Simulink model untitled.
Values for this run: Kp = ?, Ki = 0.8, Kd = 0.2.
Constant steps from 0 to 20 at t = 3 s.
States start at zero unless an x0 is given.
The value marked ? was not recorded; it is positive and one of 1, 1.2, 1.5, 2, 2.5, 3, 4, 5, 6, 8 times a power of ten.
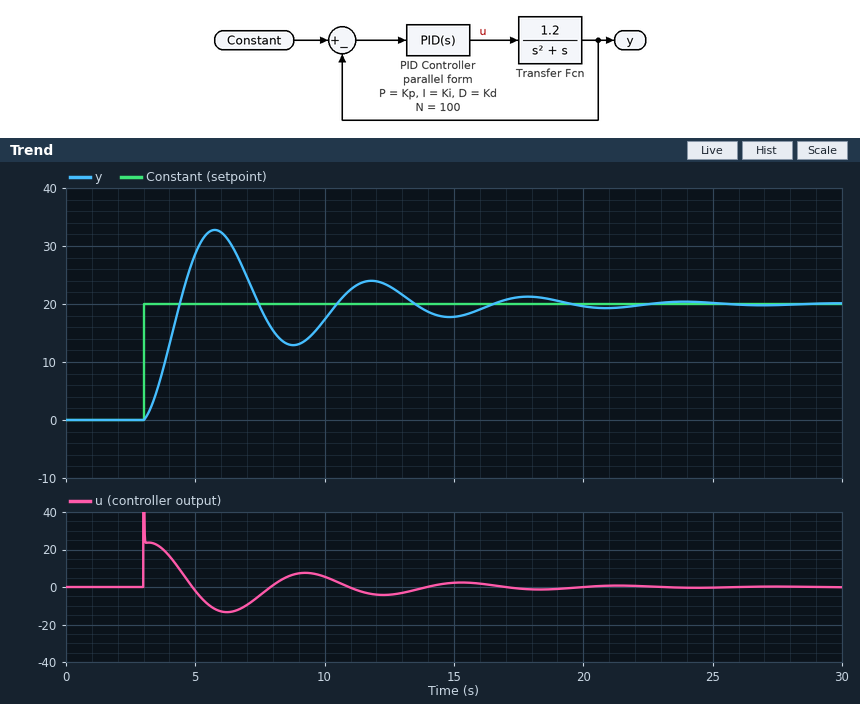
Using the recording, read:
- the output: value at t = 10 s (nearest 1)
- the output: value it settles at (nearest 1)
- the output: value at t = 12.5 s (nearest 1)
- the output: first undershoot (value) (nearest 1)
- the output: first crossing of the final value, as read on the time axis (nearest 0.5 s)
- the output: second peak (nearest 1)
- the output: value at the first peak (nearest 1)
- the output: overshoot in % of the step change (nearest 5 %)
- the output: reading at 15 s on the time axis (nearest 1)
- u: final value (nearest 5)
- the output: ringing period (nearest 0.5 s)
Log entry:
17
20
23
13
4.5 s
24
33
65 %
18
0
6.0 s
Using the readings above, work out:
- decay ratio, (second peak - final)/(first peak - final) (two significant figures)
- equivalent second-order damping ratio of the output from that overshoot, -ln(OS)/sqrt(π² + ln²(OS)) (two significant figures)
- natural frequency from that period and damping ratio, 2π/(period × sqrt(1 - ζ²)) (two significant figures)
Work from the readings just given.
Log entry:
0.31
0.14
1.1 rad/s
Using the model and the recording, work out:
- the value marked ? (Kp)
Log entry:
1.2
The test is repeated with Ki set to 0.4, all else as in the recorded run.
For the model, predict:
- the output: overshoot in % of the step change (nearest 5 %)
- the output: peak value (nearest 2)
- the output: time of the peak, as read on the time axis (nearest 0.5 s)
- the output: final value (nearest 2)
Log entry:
45 %
28
6.0 s
20
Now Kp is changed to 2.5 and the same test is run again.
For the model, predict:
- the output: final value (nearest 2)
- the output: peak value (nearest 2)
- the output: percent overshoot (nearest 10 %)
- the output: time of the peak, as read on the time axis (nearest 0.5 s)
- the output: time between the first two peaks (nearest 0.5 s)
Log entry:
20
30
50 %
5.0 s
4.0 s
